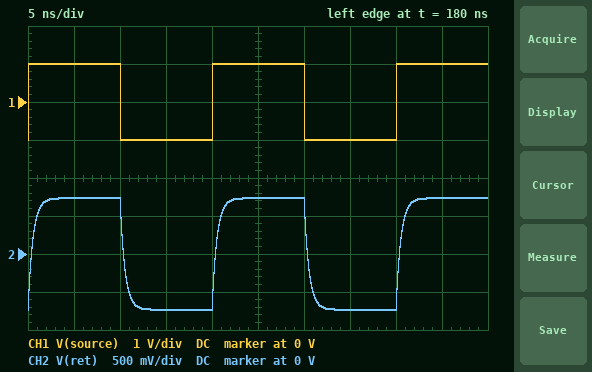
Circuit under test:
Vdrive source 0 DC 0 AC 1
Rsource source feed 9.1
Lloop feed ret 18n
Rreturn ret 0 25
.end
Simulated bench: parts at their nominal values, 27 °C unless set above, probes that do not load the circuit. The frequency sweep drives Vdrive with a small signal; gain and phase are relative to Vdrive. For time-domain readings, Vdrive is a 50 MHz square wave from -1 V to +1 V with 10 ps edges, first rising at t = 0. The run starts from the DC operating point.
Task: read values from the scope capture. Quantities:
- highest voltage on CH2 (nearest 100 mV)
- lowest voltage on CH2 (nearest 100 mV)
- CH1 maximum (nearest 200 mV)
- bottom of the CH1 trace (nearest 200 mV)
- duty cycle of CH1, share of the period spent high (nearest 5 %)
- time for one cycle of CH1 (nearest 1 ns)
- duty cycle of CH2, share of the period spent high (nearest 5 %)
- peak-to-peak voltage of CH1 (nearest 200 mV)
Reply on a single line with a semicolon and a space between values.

700 mV; -700 mV; 1.0 V; -1.0 V; 50 %; 20 ns; 50 %; 2.0 V
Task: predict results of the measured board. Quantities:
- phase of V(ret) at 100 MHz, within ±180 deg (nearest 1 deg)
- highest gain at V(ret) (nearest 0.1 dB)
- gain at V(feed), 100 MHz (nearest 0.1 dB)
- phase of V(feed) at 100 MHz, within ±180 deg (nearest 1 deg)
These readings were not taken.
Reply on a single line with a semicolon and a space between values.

-18 deg; -2.7 dB; -2.3 dB; 6 deg
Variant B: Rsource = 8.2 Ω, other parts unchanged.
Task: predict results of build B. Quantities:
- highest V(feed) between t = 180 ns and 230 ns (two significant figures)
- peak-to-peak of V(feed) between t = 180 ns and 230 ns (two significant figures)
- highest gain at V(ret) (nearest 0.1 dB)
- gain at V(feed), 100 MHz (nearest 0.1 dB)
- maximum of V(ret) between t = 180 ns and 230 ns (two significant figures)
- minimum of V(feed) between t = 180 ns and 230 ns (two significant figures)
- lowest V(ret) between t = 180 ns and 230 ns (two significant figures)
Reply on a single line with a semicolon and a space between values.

1.2 V; 2.5 V; -2.5 dB; -2.1 dB; 750 mV; -1.2 V; -750 mV
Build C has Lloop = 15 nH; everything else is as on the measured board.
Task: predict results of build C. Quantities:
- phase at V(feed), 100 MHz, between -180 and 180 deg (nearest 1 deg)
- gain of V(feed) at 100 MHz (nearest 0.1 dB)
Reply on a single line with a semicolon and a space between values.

5 deg; -2.4 dB
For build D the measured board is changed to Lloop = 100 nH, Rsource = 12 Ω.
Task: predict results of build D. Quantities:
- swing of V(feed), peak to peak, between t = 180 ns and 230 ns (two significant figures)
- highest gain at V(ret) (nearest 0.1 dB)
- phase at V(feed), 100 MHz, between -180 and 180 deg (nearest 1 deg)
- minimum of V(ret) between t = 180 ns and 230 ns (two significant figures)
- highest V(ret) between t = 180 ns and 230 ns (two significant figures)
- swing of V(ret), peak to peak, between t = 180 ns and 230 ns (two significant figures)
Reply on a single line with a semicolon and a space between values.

2.6 V; -3.4 dB; 9 deg; -640 mV; 640 mV; 1.3 V
